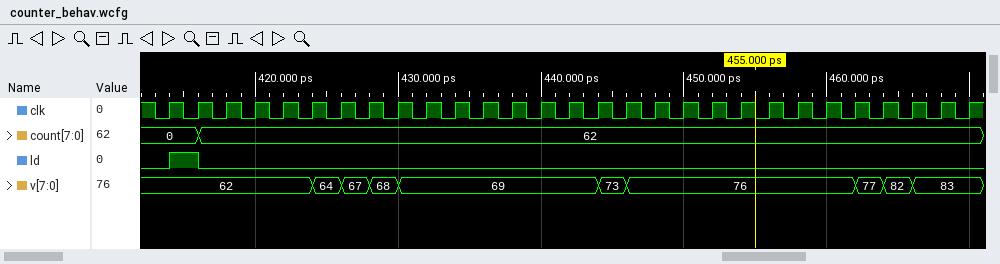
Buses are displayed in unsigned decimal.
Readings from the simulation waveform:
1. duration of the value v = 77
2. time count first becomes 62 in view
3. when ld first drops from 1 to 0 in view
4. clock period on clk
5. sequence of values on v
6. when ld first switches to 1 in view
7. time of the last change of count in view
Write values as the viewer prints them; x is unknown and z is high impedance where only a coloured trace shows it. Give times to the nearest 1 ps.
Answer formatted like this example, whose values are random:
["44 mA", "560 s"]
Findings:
["2 ps", "416 ps", "416 ps", "2 ps", "62, 64, 67, 68, 69, 73, 76, 77, 82, 83", "414 ps", "416 ps"]
